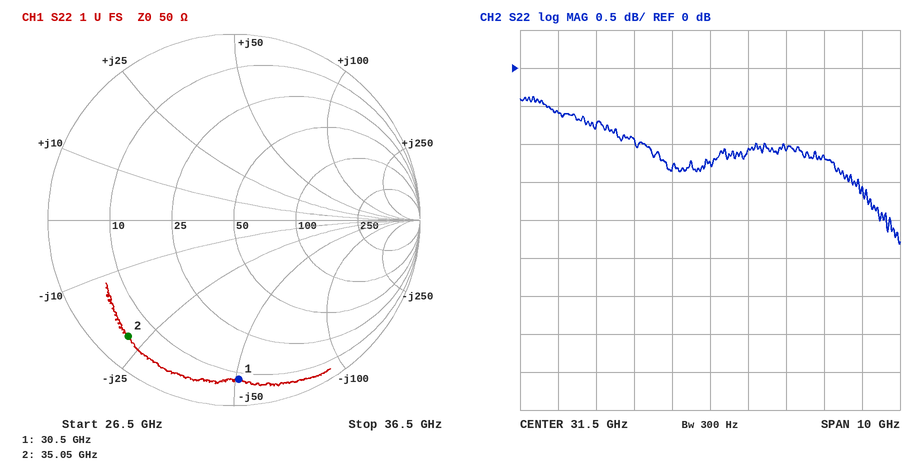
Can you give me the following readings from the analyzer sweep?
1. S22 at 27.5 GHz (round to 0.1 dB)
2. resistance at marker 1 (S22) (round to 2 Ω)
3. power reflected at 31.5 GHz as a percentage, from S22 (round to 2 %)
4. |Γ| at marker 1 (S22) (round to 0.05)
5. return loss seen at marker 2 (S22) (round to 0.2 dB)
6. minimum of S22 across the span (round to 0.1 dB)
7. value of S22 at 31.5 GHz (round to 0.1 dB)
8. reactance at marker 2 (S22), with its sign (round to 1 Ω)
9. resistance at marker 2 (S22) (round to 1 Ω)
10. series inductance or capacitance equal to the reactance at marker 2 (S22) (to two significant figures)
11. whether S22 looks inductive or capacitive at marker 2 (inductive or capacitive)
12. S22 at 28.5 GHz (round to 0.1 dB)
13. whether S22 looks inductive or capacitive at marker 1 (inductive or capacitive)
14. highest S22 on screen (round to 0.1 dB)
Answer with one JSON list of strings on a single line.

["-0.6 dB", "8 Ω", "76 %", "0.85", "1.4 dB", "-2.3 dB", "-1.2 dB", "-22 Ω", "5 Ω", "210 fF", "capacitive", "-0.8 dB", "capacitive", "-0.4 dB"]
